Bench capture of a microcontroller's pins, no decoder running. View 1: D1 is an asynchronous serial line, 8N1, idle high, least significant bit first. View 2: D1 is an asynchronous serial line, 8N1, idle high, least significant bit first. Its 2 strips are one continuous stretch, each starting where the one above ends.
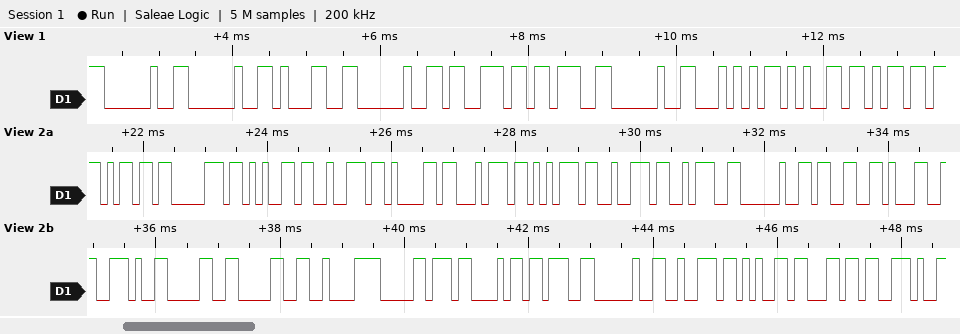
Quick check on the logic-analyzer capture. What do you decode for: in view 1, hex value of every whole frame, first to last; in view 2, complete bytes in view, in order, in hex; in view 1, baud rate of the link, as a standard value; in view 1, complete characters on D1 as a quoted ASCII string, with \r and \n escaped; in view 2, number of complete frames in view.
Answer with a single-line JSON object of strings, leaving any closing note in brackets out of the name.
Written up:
{"in view 1, hex value of every whole frame, first to last": "20 20 31 20 73 3B 20 54 65 6D", "in view 2, complete bytes in view, in order, in hex": "0x6D 0x70 0x65 0x72 0x61 0x74 0x75 0x72 0x3A 0x20 0x33 0x31 0x2E 0x30 0x30 0xC2 0xB0 0x43 0x3B 0x20 0x72 0x65 0x6C 0x2E", "in view 1, baud rate of the link, as a standard value": "9600 baud", "in view 1, complete characters on D1 as a quoted ASCII string, with \\r and \\n escaped": "\"  1 s; Tem\"", "in view 2, number of complete frames in view": "24"}
